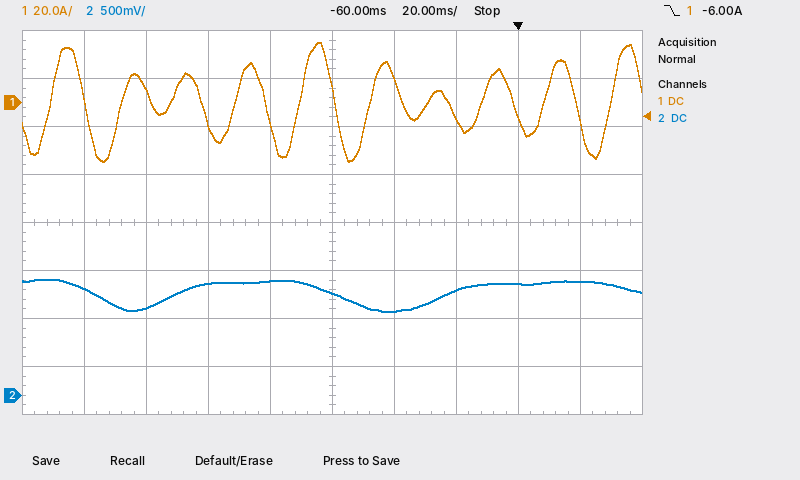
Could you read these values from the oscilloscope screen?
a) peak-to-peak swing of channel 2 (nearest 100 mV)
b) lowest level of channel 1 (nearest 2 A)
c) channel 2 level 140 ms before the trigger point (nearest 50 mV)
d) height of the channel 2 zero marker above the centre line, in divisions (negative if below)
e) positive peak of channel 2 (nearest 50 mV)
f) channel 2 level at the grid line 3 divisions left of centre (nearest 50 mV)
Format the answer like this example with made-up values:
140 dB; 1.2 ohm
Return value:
300 mV; -24 A; 1.10 V; -3.6 div; 1.20 V; 900 mV
